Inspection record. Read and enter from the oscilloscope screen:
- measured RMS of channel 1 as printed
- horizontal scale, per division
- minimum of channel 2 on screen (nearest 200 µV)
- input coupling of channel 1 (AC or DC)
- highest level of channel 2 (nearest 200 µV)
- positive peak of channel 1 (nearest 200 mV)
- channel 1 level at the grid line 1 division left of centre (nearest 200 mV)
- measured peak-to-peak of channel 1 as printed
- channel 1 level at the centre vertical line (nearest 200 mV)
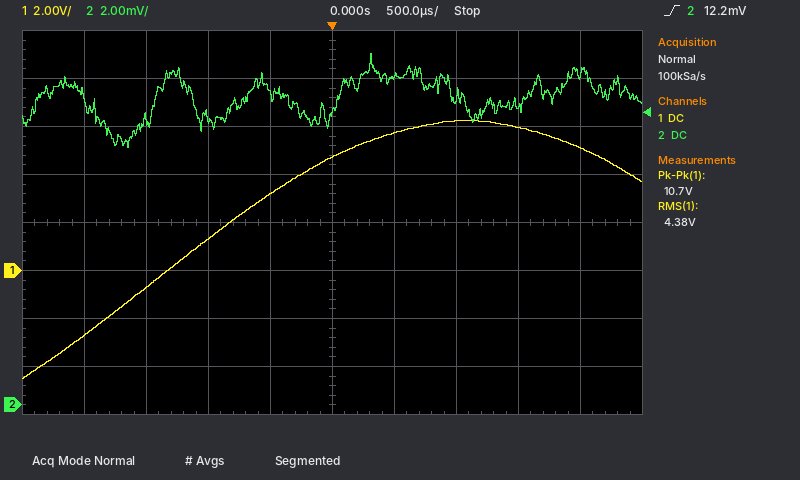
4.38 V
500 µs
10.8 mV
DC
14.6 mV
6.2 V
3.2 V
10.7 V
4.8 V
